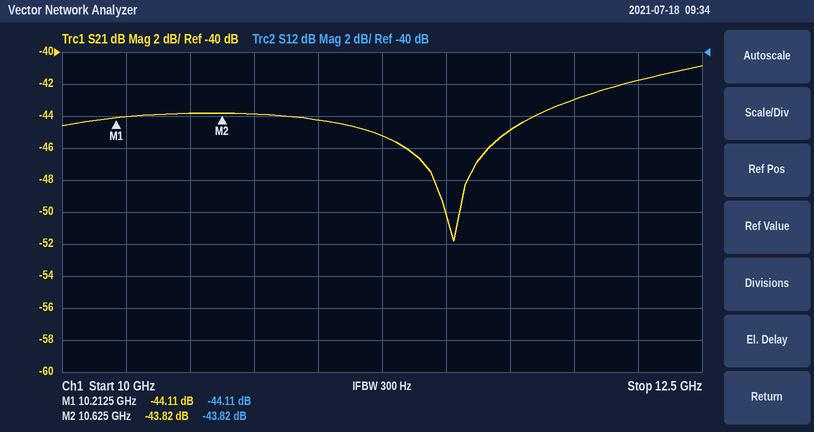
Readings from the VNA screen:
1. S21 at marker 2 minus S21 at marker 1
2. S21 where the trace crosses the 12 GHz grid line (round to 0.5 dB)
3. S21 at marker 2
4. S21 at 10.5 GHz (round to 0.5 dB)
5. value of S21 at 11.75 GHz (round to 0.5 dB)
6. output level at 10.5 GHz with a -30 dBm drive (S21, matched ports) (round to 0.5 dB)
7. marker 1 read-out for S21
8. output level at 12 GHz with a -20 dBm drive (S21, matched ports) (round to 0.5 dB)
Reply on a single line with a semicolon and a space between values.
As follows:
0.29 dB; -43.0 dB; -43.82 dB; -44.0 dB; -45.0 dB; -74.0 dBm; -44.11 dB; -63.0 dBm
